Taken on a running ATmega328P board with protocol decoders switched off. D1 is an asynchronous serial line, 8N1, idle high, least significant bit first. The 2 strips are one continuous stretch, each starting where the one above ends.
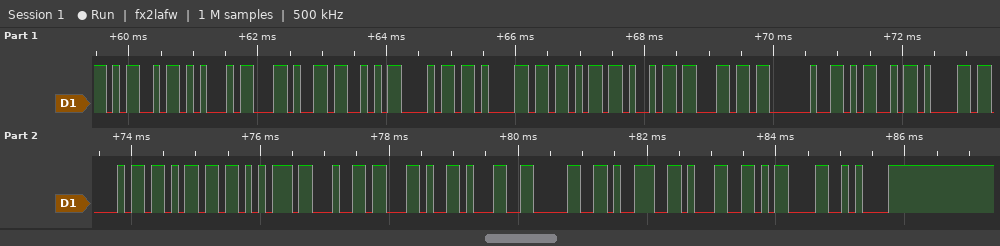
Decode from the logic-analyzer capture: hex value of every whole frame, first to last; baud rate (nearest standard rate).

4D 45 2C 53 68 61 6B 69 6C 20 4D 61 68 6D 75 64 2C 31 30 39 31 0D 0A
9600 baud
